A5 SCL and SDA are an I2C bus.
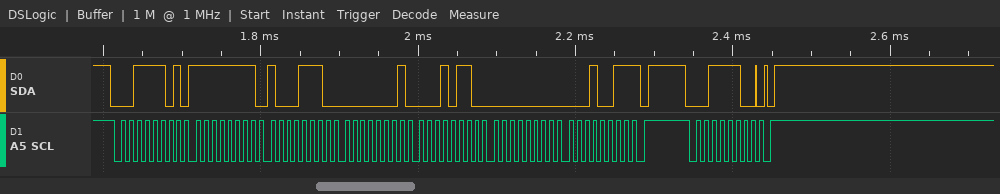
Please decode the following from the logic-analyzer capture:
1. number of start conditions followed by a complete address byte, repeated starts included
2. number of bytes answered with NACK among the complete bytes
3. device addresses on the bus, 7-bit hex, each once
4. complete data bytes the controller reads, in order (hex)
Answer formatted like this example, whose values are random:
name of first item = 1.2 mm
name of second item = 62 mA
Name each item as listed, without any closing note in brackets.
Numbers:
number of start conditions followed by a complete address byte, repeated starts included = 2
number of bytes answered with NACK among the complete bytes = 1
device addresses on the bus, 7-bit hex, each once = 0x1E
complete data bytes the controller reads, in order = FF 8E 01 16 00 13
